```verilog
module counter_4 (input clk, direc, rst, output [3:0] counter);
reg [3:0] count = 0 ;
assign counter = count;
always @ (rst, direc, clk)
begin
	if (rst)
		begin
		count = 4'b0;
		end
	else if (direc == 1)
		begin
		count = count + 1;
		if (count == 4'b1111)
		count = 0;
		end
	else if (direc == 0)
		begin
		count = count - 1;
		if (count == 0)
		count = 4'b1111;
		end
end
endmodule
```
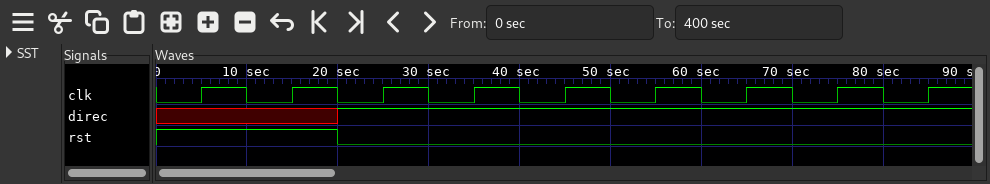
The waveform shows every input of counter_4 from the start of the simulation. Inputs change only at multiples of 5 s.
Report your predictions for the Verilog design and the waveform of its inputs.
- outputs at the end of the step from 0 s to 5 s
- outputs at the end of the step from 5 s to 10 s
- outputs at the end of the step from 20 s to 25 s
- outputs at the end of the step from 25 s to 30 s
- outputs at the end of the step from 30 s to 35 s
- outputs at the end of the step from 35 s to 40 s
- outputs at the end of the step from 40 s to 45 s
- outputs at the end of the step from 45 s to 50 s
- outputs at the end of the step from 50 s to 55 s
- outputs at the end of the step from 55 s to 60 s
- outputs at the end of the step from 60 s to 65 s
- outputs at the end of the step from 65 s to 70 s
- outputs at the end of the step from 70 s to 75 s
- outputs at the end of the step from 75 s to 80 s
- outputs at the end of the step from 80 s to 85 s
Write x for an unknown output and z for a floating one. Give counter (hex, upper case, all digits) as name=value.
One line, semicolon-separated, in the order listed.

counter=0; counter=0; counter=1; counter=2; counter=3; counter=4; counter=5; counter=6; counter=7; counter=8; counter=9; counter=A; counter=B; counter=C; counter=D
